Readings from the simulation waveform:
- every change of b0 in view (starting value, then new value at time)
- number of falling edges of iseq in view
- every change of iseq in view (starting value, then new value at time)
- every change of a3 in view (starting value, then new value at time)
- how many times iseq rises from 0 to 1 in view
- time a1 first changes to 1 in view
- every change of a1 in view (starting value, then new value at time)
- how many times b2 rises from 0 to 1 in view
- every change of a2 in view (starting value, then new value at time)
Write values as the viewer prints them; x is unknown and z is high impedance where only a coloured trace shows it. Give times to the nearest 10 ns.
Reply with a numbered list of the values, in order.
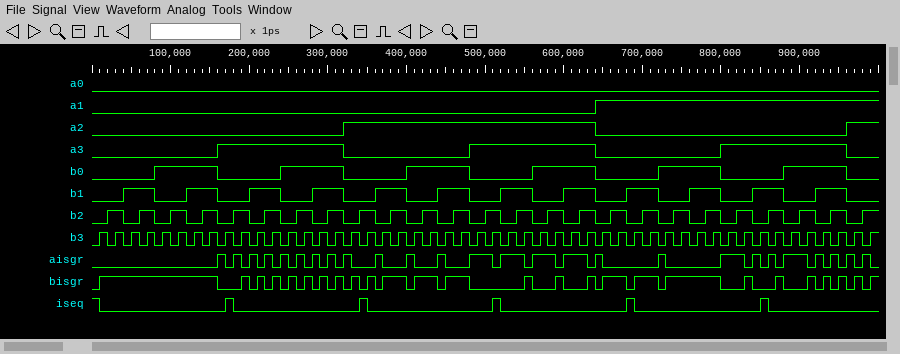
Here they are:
1. 0, 1 at 80 ns, 0 at 160 ns, 1 at 240 ns, 0 at 320 ns, 1 at 400 ns, 0 at 480 ns, 1 at 560 ns, 0 at 640 ns, 1 at 720 ns, 0 at 800 ns, 1 at 880 ns, 0 at 960 ns
2. 6
3. 1, 0 at 10 ns, 1 at 170 ns, 0 at 180 ns, 1 at 340 ns, 0 at 350 ns, 1 at 510 ns, 0 at 520 ns, 1 at 680 ns, 0 at 690 ns, 1 at 850 ns, 0 at 860 ns
4. 0, 1 at 160 ns, 0 at 320 ns, 1 at 480 ns, 0 at 640 ns, 1 at 800 ns, 0 at 960 ns
5. 5
6. 640 ns
7. 0, 1 at 640 ns
8. 25
9. 0, 1 at 320 ns, 0 at 640 ns, 1 at 960 ns
